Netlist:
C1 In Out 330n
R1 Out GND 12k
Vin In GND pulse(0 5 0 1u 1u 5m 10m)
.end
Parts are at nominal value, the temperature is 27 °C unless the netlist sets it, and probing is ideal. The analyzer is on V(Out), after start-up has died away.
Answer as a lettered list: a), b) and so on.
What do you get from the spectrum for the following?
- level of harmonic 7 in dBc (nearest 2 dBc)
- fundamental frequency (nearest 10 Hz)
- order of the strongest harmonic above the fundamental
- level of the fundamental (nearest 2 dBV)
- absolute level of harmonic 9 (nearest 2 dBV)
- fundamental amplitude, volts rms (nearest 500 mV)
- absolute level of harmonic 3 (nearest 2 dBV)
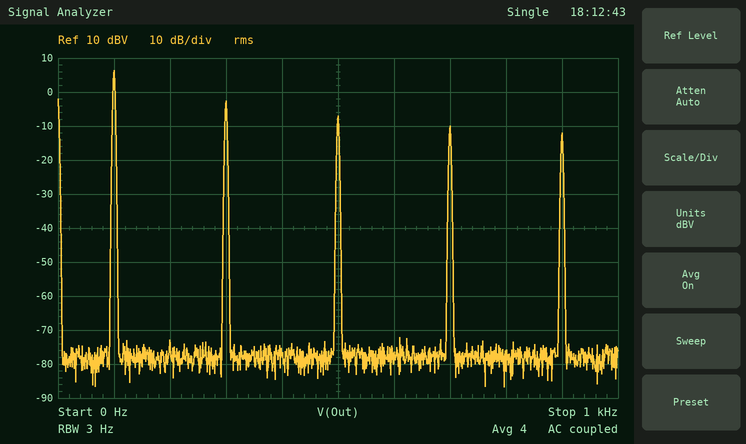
a) -16 dBc
b) 100 Hz
c) 3
d) 6 dBV
e) -12 dBV
f) 2.0 V
g) -2 dBV
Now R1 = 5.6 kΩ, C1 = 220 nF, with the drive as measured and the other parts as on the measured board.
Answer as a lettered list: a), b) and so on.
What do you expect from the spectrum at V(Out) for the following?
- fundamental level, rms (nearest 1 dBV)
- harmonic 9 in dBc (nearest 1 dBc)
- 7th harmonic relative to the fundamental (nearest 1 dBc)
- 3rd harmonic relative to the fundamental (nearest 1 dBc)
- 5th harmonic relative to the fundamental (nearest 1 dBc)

a) 3 dBV
b) -15 dBc
c) -13 dBc
d) -6 dBc
e) -10 dBc
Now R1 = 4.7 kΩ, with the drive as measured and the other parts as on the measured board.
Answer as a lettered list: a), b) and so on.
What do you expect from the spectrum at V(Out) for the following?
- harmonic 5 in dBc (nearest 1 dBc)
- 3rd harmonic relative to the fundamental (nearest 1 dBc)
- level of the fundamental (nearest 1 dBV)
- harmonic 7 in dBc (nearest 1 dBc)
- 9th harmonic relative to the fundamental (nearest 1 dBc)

a) -11 dBc
b) -7 dBc
c) 4 dBV
d) -14 dBc
e) -16 dBc
